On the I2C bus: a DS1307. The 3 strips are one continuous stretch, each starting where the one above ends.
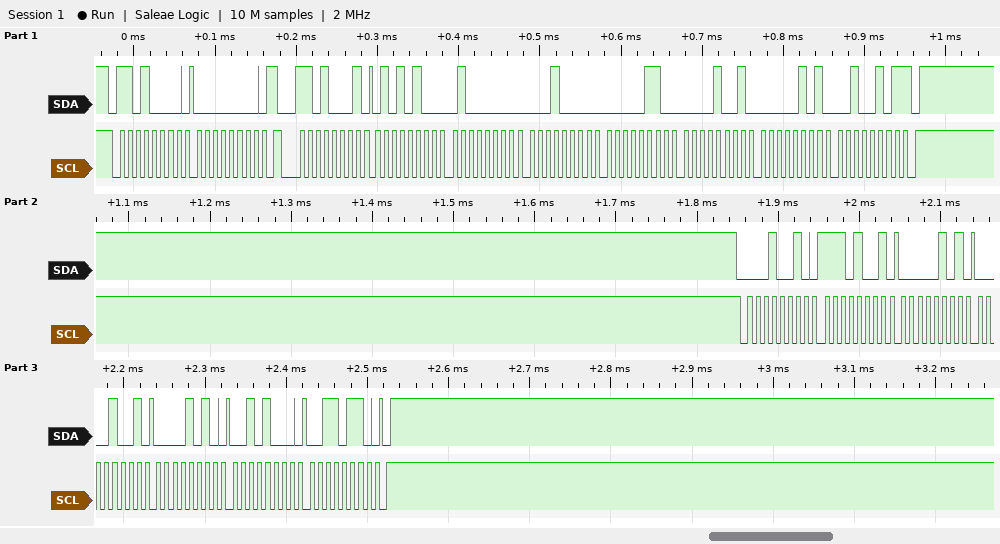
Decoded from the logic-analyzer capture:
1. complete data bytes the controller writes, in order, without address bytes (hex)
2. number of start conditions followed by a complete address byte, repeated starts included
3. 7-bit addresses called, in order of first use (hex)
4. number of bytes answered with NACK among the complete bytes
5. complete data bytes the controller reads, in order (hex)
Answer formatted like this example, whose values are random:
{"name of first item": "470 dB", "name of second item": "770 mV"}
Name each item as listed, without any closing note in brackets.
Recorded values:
{"complete data bytes the controller writes, in order, without address bytes": "00 E9 05 09 0A 28 36", "number of start conditions followed by a complete address byte, repeated starts included": "3", "7-bit addresses called, in order of first use": "0x68 0x09", "number of bytes answered with NACK among the complete bytes": "1", "complete data bytes the controller reads, in order": "54 40 10 06 09 05 25"}
